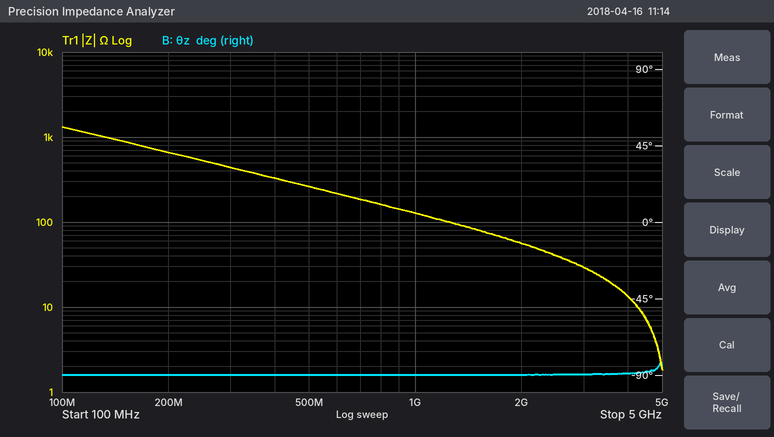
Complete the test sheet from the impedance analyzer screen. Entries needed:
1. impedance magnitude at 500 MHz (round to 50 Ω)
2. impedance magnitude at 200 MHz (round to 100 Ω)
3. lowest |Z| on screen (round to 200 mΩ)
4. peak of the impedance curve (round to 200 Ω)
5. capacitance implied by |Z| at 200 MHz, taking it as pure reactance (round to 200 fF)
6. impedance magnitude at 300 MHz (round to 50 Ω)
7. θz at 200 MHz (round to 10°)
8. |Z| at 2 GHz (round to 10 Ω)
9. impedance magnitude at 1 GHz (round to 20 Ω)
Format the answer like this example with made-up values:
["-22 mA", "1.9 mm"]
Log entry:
["250 Ω", "700 Ω", "1.8 Ω", "1.4 kΩ", "1.2 pF", "450 Ω", "-90°", "60 Ω", "120 Ω"]
